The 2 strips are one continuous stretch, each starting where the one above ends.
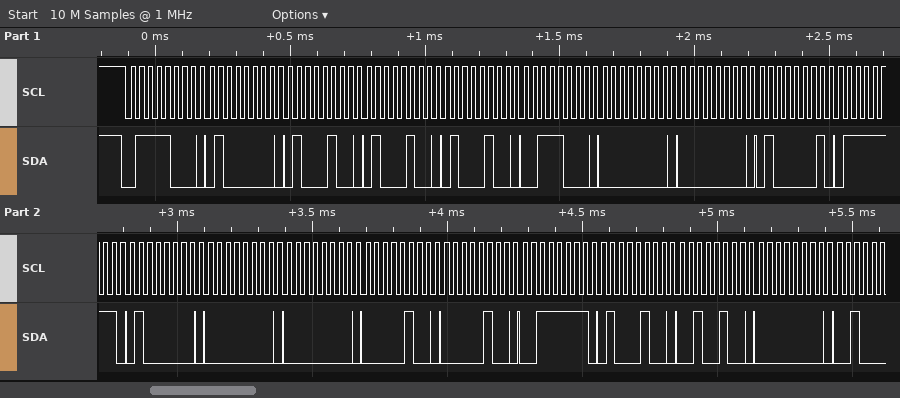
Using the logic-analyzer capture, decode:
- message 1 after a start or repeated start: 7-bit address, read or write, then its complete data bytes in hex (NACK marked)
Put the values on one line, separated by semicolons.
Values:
0x3C write: 40 44 44 44 38 00 00 41 7F 40 00 00 04 04 3F 44 24 00
